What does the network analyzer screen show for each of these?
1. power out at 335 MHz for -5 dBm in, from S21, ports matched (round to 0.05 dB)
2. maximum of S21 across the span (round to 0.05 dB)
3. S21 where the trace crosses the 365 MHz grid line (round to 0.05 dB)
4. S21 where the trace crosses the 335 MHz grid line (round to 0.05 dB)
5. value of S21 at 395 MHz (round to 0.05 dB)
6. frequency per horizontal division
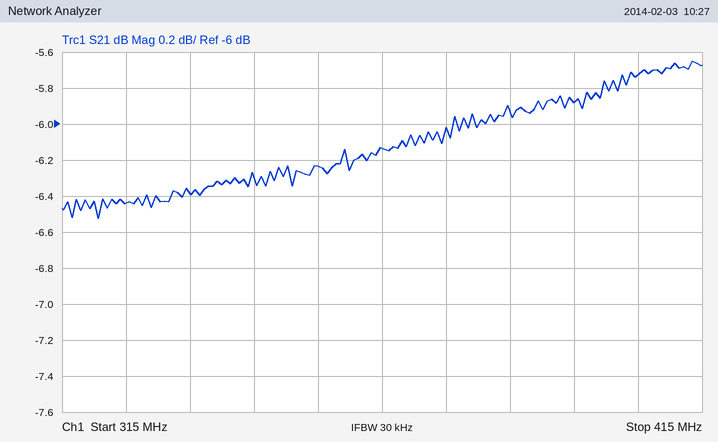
-11.40 dBm
-5.65 dB
-6.15 dB
-6.40 dB
-5.90 dB
10 MHz
